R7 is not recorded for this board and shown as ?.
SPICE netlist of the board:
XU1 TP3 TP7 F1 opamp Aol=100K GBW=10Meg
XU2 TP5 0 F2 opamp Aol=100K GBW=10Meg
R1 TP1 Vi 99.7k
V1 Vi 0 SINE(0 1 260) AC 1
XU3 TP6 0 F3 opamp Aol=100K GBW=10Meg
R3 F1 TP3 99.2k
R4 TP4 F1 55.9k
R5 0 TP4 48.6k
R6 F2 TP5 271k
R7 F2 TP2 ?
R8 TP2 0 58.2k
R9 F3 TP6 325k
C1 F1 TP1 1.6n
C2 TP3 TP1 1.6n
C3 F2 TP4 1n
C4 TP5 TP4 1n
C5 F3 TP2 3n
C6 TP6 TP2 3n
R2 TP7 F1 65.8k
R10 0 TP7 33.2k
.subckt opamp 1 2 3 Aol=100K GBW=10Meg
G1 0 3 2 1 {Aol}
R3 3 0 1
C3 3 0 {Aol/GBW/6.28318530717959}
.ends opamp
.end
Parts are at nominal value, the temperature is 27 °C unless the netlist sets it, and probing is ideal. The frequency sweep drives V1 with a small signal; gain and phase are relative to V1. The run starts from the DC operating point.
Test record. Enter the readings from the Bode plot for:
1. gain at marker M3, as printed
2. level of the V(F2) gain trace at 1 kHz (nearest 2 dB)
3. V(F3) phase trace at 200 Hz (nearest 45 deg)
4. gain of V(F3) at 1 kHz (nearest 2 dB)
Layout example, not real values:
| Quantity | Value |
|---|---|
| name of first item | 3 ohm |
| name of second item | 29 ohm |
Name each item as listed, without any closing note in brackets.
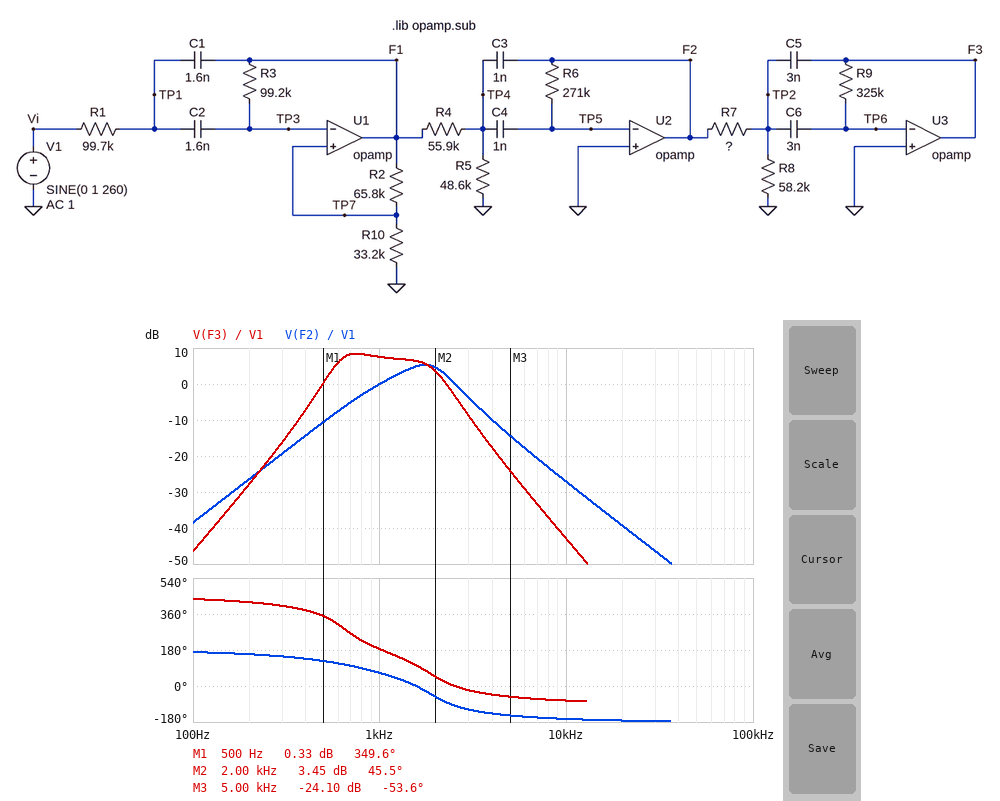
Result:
| Quantity | Value |
|---|---|
| gain at marker M3, as printed | -24.10 dB |
| level of the V(F2) gain trace at 1 kHz | 0 dB |
| V(F3) phase trace at 200 Hz | 405 deg |
| gain of V(F3) at 1 kHz | 8 dB |
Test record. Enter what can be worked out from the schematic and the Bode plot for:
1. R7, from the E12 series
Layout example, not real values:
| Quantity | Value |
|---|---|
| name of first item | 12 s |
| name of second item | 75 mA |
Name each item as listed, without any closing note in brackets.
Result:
| Quantity | Value |
|---|---|
| R7, from the E12 series | 33 kΩ |
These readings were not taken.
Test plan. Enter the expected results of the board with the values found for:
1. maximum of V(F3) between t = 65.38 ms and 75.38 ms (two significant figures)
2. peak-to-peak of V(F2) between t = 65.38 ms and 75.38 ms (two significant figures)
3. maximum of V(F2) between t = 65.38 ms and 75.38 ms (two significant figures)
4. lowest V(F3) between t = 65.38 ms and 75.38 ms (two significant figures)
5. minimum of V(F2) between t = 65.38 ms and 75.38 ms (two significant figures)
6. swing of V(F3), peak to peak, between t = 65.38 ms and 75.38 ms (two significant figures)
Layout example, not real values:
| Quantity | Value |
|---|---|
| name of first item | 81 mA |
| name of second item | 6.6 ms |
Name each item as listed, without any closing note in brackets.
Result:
| Quantity | Value |
|---|---|
| maximum of V(F3) between t = 65.38 ms and 75.38 ms | 95 mV |
| peak-to-peak of V(F2) between t = 65.38 ms and 75.38 ms | 160 mV |
| maximum of V(F2) between t = 65.38 ms and 75.38 ms | 81 mV |
| lowest V(F3) between t = 65.38 ms and 75.38 ms | -95 mV |
| minimum of V(F2) between t = 65.38 ms and 75.38 ms | -81 mV |
| swing of V(F3), peak to peak, between t = 65.38 ms and 75.38 ms | 190 mV |
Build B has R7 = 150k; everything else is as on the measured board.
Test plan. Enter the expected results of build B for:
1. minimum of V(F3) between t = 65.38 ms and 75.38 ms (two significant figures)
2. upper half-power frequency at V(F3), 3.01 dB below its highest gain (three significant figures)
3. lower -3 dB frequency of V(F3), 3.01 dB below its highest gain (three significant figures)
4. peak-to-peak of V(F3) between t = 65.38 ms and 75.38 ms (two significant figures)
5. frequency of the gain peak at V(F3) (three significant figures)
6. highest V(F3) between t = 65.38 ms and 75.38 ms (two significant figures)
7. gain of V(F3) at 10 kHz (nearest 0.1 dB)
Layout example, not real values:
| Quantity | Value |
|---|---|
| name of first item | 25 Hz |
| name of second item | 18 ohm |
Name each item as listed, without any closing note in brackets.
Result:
| Quantity | Value |
|---|---|
| minimum of V(F3) between t = 65.38 ms and 75.38 ms | -46 mV |
| upper half-power frequency at V(F3), 3.01 dB below its highest gain | 2.02 kHz |
| lower -3 dB frequency of V(F3), 3.01 dB below its highest gain | 490 Hz |
| peak-to-peak of V(F3) between t = 65.38 ms and 75.38 ms | 91 mV |
| frequency of the gain peak at V(F3) | 1.40 kHz |
| highest V(F3) between t = 65.38 ms and 75.38 ms | 46 mV |
| gain of V(F3) at 10 kHz | -56.2 dB |
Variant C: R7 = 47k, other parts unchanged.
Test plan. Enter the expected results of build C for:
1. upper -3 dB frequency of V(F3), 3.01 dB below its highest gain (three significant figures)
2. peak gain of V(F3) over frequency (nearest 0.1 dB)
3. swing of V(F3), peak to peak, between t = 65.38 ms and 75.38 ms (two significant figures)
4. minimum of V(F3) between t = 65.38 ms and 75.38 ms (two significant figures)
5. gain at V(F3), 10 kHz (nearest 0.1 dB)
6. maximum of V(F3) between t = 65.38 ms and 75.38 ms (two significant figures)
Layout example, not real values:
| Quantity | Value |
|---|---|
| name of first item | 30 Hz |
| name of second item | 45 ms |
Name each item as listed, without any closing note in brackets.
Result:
| Quantity | Value |
|---|---|
| upper -3 dB frequency of V(F3), 3.01 dB below its highest gain | 1.92 kHz |
| peak gain of V(F3) over frequency | 4.0 dB |
| swing of V(F3), peak to peak, between t = 65.38 ms and 75.38 ms | 170 mV |
| minimum of V(F3) between t = 65.38 ms and 75.38 ms | -85 mV |
| gain at V(F3), 10 kHz | -46.1 dB |
| maximum of V(F3) between t = 65.38 ms and 75.38 ms | 85 mV |
